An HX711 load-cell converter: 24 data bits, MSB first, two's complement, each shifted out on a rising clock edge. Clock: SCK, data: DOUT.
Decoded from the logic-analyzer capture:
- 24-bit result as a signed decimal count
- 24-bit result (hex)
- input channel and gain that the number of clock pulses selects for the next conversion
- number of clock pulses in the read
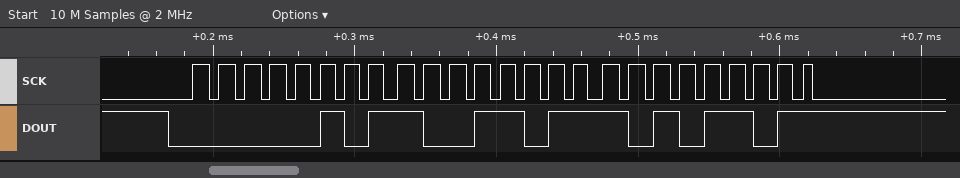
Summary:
367533
0x059BAD
channel A, gain 128
25
